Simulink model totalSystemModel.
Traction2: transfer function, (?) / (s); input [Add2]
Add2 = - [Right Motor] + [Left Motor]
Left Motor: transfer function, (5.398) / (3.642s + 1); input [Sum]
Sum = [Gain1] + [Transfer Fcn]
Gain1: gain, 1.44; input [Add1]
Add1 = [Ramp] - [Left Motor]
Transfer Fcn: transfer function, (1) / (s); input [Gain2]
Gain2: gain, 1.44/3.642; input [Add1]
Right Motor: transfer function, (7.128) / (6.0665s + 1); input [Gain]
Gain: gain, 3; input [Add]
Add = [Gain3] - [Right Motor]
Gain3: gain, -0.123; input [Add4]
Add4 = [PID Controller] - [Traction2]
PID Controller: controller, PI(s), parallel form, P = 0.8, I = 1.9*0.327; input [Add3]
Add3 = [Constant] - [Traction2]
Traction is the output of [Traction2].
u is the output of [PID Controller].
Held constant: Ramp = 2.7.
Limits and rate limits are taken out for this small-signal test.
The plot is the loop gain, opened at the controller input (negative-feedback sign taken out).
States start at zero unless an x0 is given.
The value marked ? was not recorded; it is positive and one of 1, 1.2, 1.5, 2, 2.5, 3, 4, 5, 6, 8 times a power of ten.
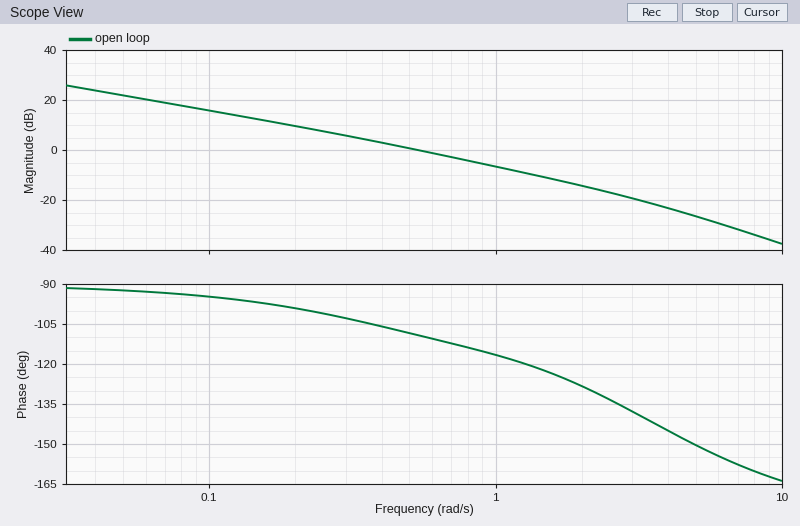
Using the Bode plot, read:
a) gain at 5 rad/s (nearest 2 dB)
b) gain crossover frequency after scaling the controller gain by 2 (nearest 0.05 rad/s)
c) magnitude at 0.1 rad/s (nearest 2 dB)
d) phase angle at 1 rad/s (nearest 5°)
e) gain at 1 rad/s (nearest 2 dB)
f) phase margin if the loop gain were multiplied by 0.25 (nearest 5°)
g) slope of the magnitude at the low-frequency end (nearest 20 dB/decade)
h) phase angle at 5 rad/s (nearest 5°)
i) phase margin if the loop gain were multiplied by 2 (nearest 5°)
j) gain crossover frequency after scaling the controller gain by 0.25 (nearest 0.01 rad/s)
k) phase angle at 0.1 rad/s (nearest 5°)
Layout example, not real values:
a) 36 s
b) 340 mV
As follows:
a) -26 dB
b) 0.95 rad/s
c) 16 dB
d) -115°
e) -6 dB
f) 85°
g) -20 dB/decade
h) -150°
i) 65°
j) 0.15 rad/s
k) -95°
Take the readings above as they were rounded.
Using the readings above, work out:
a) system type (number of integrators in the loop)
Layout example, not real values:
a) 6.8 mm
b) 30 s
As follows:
a) 1
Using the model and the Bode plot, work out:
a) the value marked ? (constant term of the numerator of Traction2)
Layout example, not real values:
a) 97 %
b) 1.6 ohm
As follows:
a) 4
